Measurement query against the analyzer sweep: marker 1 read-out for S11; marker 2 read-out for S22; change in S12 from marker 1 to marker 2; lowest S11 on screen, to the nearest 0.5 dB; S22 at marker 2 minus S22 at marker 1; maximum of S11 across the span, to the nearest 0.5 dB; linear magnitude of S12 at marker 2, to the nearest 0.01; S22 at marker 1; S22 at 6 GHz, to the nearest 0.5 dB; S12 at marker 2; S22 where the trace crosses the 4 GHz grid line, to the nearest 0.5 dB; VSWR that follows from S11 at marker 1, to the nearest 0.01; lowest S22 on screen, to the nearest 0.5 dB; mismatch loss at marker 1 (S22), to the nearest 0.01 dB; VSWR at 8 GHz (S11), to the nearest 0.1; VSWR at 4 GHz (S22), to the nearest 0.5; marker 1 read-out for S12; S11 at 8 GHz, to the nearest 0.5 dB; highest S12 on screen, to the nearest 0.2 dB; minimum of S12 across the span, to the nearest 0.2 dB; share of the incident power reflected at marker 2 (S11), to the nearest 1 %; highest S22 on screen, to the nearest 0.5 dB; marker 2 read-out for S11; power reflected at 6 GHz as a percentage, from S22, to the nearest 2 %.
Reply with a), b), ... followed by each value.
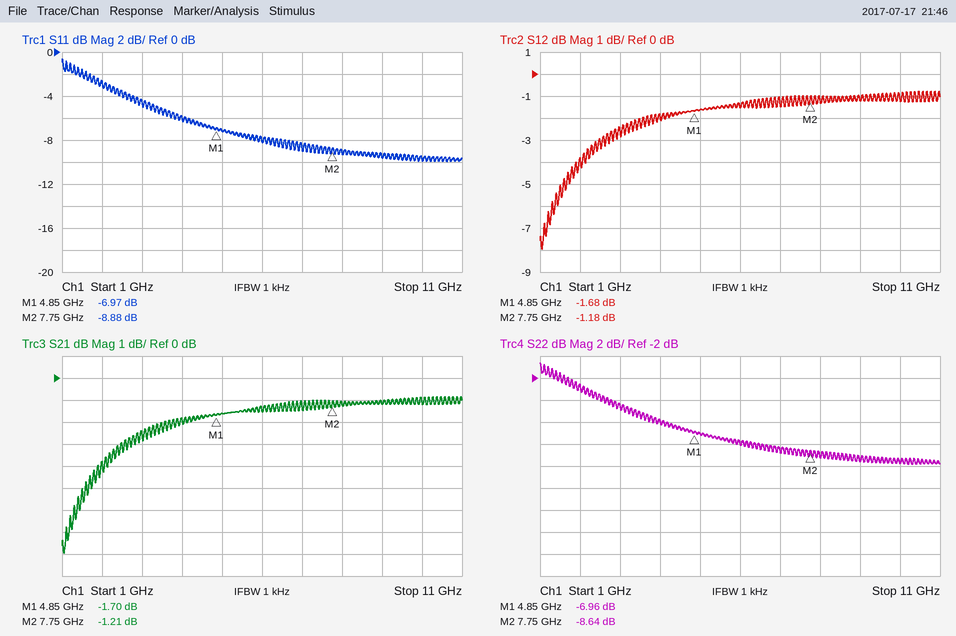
a) -6.97 dB
b) -8.64 dB
c) 0.50 dB
d) -10.0 dB
e) -1.68 dB
f) -0.5 dB
g) 0.87
h) -6.96 dB
i) -8.0 dB
j) -1.18 dB
k) -6.0 dB
l) 2.62
m) -10.0 dB
n) 0.98 dB
o) 2.1
p) 3.0
q) -1.68 dB
r) -9.0 dB
s) -0.8 dB
t) -8.0 dB
u) 13 %
v) -0.5 dB
w) -8.88 dB
x) 16 %
